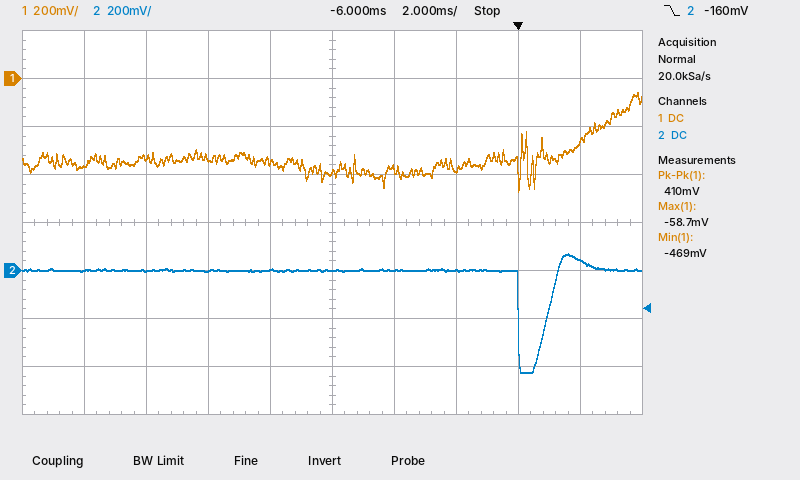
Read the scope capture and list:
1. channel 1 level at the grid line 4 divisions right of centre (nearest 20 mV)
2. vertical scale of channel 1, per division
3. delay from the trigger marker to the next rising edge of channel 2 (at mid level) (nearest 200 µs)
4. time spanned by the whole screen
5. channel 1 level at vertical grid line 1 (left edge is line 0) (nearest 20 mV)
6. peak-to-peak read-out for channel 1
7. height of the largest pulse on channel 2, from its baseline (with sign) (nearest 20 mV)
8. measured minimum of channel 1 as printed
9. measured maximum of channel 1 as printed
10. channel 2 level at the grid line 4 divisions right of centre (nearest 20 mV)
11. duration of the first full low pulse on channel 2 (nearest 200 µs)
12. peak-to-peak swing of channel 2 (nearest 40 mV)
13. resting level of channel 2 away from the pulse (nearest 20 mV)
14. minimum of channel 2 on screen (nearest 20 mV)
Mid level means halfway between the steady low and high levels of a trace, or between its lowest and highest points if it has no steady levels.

-260 mV
200 mV
1.0 ms
20 ms
-360 mV
410 mV
-420 mV
-469 mV
-58.7 mV
40 mV
1.0 ms
480 mV
0 mV
-420 mV
